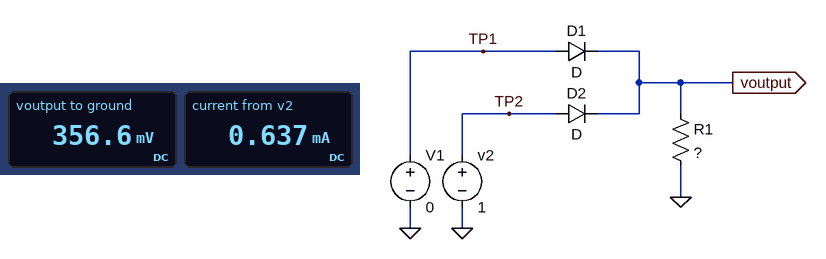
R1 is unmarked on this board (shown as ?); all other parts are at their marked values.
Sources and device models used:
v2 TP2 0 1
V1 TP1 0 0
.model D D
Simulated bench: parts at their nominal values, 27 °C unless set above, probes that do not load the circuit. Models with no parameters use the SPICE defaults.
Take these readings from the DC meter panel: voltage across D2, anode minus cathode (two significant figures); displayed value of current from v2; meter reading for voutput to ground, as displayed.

640 mV
0.637 mA
356.6 mV
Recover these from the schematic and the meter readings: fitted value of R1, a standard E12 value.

560 Ω
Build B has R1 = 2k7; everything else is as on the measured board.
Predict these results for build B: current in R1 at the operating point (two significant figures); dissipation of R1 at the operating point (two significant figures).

150 µA
58 µW
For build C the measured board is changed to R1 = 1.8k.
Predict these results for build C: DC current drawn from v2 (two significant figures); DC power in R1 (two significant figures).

210 µA
82 µW
